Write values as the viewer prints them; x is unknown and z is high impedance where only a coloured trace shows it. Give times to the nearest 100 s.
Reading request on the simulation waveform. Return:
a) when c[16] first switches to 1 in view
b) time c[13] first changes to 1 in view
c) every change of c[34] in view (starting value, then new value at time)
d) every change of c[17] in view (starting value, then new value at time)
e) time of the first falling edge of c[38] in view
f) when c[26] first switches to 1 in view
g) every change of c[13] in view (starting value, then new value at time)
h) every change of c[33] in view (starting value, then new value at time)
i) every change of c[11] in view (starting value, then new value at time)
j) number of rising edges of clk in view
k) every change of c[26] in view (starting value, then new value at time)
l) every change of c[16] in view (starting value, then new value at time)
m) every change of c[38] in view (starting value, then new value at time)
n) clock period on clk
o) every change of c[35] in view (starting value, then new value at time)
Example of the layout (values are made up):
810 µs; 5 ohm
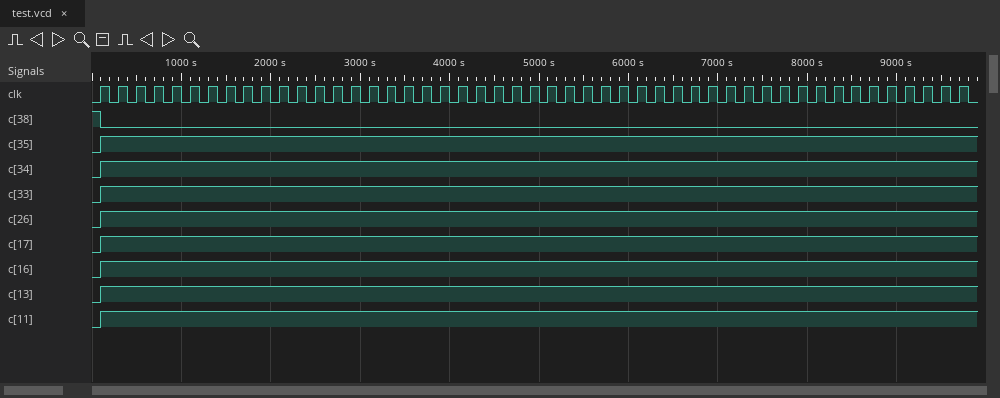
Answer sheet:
100 s; 100 s; 0, 1 at 100 s; 0, 1 at 100 s; 100 s; 100 s; 0, 1 at 100 s; 0, 1 at 100 s; 0, 1 at 100 s; 49; 0, 1 at 100 s; 0, 1 at 100 s; 1, 0 at 100 s; 200 s; 0, 1 at 100 s
